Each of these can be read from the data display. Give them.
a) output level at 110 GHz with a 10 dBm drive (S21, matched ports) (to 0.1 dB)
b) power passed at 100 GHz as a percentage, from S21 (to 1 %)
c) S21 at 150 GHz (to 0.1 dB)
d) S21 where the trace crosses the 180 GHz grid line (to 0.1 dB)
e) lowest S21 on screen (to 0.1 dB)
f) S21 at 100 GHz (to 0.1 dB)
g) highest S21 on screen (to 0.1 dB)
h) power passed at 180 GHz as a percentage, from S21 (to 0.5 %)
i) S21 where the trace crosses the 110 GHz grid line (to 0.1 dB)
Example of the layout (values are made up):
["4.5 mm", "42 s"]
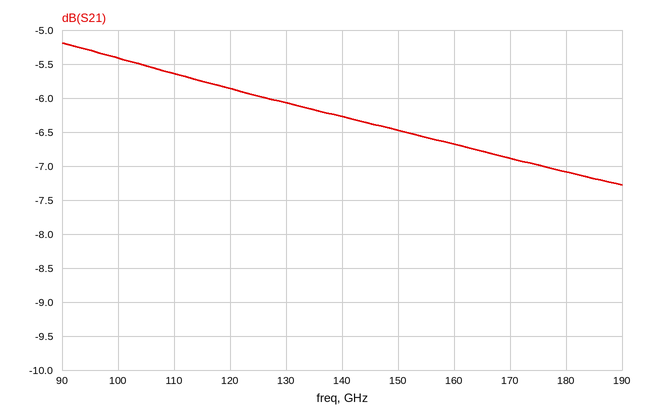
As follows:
["4.4 dBm", "29 %", "-6.5 dB", "-7.1 dB", "-7.3 dB", "-5.4 dB", "-5.2 dB", "19.5 %", "-5.6 dB"]
